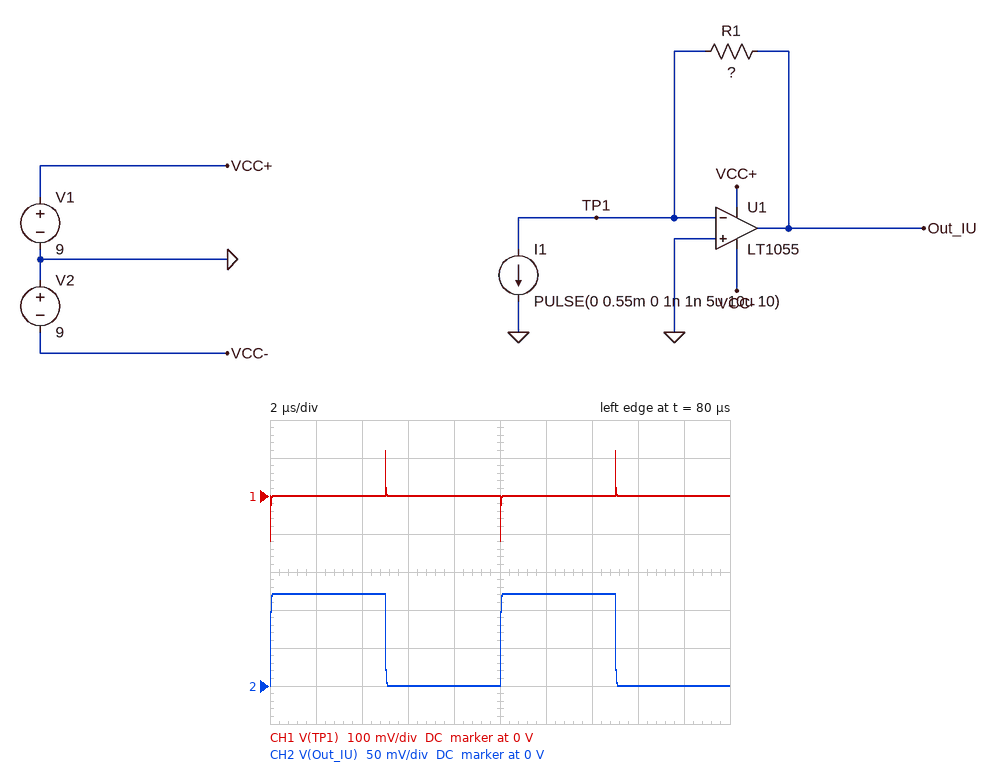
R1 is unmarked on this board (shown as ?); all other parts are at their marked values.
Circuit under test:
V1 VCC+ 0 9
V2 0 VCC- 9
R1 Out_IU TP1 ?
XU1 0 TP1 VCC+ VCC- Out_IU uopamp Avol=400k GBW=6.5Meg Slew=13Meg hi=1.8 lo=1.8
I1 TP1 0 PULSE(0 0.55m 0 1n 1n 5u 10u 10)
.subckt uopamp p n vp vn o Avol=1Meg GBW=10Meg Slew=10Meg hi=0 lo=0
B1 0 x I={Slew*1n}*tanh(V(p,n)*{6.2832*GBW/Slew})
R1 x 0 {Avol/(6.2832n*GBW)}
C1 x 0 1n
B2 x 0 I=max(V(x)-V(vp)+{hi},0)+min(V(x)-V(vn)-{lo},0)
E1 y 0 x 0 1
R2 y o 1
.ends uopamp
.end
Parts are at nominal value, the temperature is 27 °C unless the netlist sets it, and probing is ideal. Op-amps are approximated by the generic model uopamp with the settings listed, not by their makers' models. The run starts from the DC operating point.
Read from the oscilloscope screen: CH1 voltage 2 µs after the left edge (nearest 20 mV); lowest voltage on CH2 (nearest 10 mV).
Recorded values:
0 V
0 V
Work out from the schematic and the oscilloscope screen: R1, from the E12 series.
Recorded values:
220 Ω
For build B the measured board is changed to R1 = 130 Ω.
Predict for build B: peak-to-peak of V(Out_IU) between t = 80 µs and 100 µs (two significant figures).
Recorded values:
72 mV
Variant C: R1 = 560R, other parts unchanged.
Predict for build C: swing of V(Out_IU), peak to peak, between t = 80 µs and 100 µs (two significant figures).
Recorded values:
310 mV
